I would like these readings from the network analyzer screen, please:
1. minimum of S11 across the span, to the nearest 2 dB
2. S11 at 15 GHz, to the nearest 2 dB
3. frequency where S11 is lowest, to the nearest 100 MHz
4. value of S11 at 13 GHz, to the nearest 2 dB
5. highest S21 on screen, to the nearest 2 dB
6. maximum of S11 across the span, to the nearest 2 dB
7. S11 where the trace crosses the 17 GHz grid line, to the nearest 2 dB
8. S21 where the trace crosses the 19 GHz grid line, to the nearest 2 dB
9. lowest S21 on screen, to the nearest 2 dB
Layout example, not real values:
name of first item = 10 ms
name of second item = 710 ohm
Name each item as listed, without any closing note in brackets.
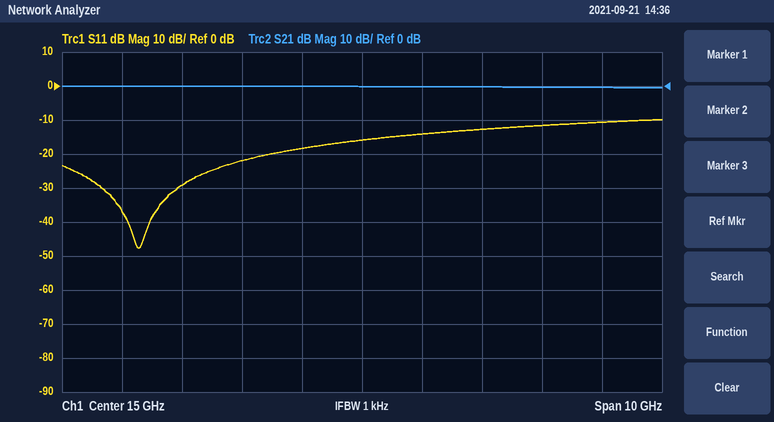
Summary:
minimum of S11 across the span, to the nearest 2 dB = -48 dB
S11 at 15 GHz, to the nearest 2 dB = -16 dB
frequency where S11 is lowest, to the nearest 100 MHz = 11.3 GHz
value of S11 at 13 GHz, to the nearest 2 dB = -22 dB
highest S21 on screen, to the nearest 2 dB = 0 dB
maximum of S11 across the span, to the nearest 2 dB = -10 dB
S11 where the trace crosses the 17 GHz grid line, to the nearest 2 dB = -12 dB
S21 where the trace crosses the 19 GHz grid line, to the nearest 2 dB = 0 dB
lowest S21 on screen, to the nearest 2 dB = 0 dB
